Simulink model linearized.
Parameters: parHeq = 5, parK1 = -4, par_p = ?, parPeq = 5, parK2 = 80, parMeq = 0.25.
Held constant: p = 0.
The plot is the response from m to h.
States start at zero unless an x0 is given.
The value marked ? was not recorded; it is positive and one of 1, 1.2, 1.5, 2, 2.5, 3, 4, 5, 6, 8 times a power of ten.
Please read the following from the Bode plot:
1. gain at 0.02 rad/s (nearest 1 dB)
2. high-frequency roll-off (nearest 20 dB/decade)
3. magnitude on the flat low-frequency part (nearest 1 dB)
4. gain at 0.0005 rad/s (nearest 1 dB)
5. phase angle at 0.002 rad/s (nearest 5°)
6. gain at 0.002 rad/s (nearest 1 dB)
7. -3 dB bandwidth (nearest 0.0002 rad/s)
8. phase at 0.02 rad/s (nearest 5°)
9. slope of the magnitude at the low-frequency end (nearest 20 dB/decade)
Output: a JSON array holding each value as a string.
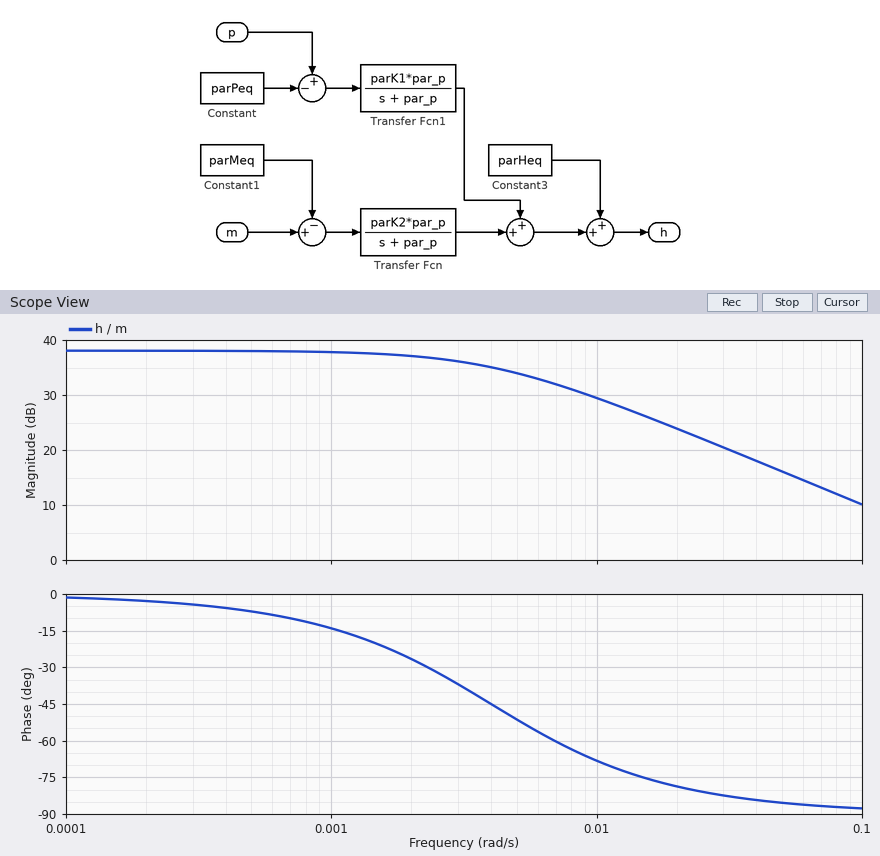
["24 dB", "-20 dB/decade", "38 dB", "38 dB", "-25°", "37 dB", "0.0040 rad/s", "-80°", "0 dB/decade"]
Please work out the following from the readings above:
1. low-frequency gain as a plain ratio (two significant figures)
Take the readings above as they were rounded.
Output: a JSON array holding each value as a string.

["79"]
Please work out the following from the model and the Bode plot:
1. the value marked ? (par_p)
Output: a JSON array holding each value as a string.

["0.004"]
